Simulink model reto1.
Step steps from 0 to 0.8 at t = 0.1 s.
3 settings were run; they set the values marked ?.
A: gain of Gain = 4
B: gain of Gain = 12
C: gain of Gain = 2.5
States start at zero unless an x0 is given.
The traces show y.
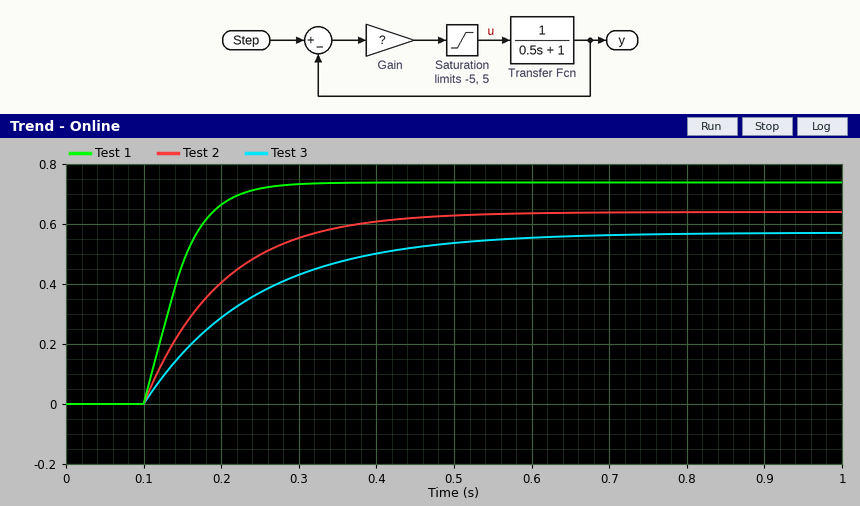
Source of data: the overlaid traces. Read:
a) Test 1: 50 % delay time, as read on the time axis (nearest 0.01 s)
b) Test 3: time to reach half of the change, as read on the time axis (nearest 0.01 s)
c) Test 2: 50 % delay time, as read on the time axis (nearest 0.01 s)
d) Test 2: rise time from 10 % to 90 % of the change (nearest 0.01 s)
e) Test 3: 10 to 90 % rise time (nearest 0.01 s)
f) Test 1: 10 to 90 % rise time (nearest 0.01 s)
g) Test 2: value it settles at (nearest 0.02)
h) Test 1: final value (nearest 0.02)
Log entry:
0.14 s
0.20 s
0.17 s
0.22 s
0.31 s
0.09 s
0.64
0.74
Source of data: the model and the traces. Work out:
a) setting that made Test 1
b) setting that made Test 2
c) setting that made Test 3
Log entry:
B
A
C
